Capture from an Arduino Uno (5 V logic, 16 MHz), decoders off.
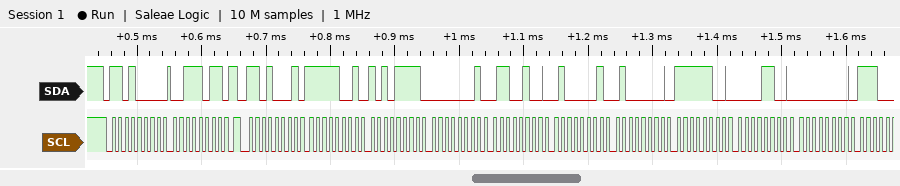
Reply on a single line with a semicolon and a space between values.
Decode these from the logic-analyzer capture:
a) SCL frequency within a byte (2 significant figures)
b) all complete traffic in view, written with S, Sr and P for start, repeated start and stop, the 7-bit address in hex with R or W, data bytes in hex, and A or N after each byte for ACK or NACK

100 kHz; S 68W A 3B A Sr 68R A F9 A AF A 01 A 64 A 41 A 40 A FC A 0C A 00 A
